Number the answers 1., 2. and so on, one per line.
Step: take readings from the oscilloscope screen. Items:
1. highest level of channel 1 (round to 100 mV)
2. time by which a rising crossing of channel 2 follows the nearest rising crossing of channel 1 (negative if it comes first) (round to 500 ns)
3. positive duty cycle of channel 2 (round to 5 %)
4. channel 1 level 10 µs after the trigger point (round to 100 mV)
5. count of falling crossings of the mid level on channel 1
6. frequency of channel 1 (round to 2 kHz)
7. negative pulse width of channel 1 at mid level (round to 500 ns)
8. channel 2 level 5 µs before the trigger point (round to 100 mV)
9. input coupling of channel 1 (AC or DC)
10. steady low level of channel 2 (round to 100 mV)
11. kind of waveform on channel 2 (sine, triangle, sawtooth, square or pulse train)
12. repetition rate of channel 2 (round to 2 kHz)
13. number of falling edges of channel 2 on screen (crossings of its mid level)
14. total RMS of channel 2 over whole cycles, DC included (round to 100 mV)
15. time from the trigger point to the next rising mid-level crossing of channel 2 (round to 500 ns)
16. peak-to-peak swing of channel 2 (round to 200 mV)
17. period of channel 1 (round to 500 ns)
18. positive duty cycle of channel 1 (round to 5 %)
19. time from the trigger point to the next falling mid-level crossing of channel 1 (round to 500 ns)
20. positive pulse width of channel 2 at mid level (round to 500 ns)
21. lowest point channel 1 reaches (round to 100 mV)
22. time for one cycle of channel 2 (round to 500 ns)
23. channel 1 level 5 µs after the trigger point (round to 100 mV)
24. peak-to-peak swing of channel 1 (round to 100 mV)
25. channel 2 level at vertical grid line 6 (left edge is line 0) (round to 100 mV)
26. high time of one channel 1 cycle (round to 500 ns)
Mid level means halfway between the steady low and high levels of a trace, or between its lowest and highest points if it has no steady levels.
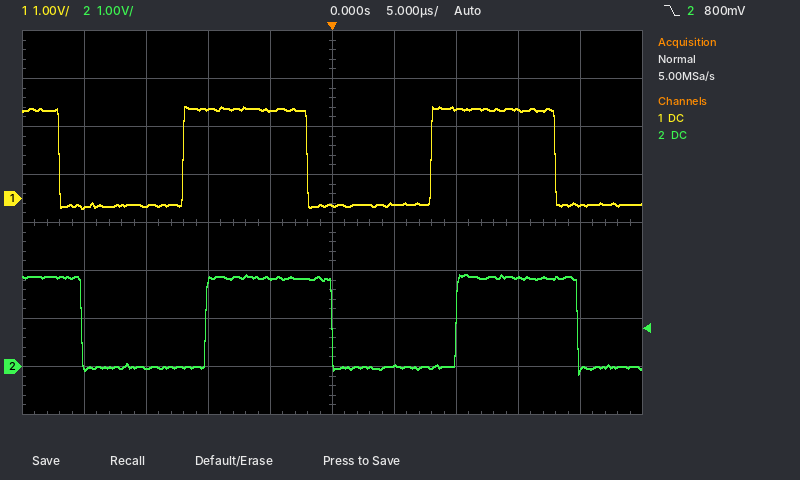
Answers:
1. 1.9 V
2. +2.0 µs
3. 50 %
4. 1.9 V
5. 3
6. 50 kHz
7. 10.0 µs
8. 1.8 V
9. DC
10. 0.0 V
11. square
12. 50 kHz
13. 3
14. 1.3 V
15. 10.0 µs
16. 2.0 V
17. 20.0 µs
18. 50 %
19. 18.0 µs
20. 10.0 µs
21. -200 mV
22. 20.0 µs
23. -100 mV
24. 2.1 V
25. 0.0 V
26. 10.0 µs
